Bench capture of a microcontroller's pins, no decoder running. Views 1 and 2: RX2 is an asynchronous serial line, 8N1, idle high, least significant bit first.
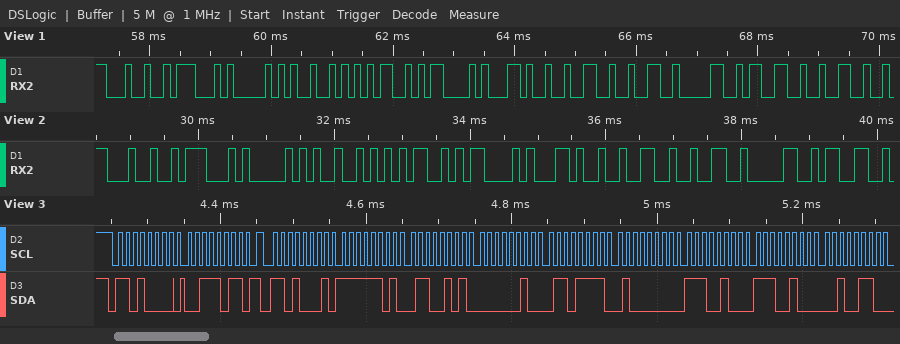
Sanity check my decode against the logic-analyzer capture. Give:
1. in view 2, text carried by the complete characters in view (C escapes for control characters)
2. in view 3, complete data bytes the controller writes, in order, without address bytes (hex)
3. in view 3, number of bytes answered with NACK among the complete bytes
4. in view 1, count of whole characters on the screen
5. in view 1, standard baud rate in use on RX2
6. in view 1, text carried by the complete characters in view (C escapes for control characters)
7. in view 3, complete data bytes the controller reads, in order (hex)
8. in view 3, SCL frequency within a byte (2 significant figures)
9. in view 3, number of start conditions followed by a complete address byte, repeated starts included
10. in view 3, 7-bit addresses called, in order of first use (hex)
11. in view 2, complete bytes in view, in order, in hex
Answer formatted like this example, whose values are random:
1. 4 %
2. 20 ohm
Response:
1. "$GPRMC,2203"
2. 3B
3. 0
4. 12
5. 9600 baud
6. "$GPRMC,22032"
7. FD 65 02 6F 40 E4 E4 26
8. 100 kHz
9. 2
10. 0x68
11. 24 47 50 52 4D 43 2C 32 32 30 33
